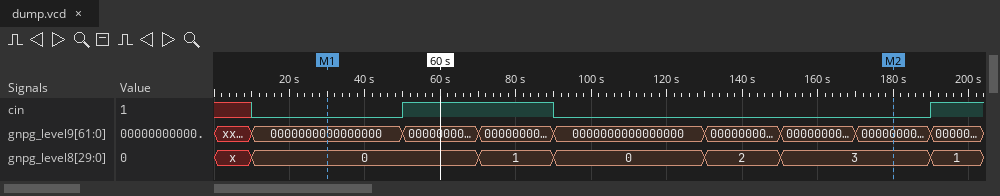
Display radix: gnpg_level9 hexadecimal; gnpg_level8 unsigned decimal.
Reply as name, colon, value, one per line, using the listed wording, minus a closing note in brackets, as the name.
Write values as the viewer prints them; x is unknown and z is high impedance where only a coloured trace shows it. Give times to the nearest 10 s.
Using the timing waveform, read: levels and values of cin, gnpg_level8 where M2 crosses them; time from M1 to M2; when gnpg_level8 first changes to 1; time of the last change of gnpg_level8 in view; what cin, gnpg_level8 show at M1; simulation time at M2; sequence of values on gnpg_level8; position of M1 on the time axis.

levels and values of cin, gnpg_level8 where M2 crosses them: cin=0, gnpg_level8=3
time from M1 to M2: 150 s
when gnpg_level8 first changes to 1: 70 s
time of the last change of gnpg_level8 in view: 190 s
what cin, gnpg_level8 show at M1: cin=0, gnpg_level8=0
simulation time at M2: 180 s
sequence of values on gnpg_level8: x, 0, 1, 0, 2, 3, 1
position of M1 on the time axis: 30 s
